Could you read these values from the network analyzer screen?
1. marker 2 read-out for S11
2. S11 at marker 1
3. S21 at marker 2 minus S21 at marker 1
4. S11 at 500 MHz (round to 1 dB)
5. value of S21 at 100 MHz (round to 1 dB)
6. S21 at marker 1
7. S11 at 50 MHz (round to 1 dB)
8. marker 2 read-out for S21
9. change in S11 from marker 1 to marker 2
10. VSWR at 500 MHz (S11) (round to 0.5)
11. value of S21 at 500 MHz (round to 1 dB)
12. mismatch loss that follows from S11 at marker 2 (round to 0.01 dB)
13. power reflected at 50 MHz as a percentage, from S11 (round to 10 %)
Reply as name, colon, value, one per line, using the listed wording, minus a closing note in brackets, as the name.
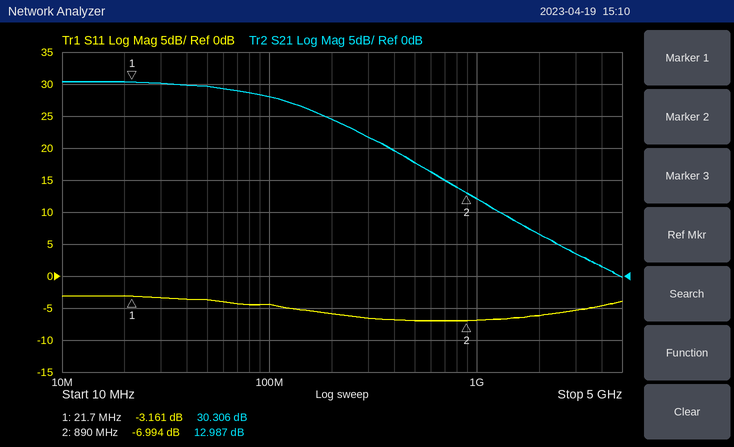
marker 2 read-out for S11: -6.994 dB
S11 at marker 1: -3.161 dB
S21 at marker 2 minus S21 at marker 1: -17.319 dB
S11 at 500 MHz: -7 dB
value of S21 at 100 MHz: 28 dB
S21 at marker 1: 30.306 dB
S11 at 50 MHz: -4 dB
marker 2 read-out for S21: 12.987 dB
change in S11 from marker 1 to marker 2: -3.833 dB
VSWR at 500 MHz (S11): 2.5
value of S21 at 500 MHz: 18 dB
mismatch loss that follows from S11 at marker 2: 0.97 dB
power reflected at 50 MHz as a percentage, from S11: 40 %
